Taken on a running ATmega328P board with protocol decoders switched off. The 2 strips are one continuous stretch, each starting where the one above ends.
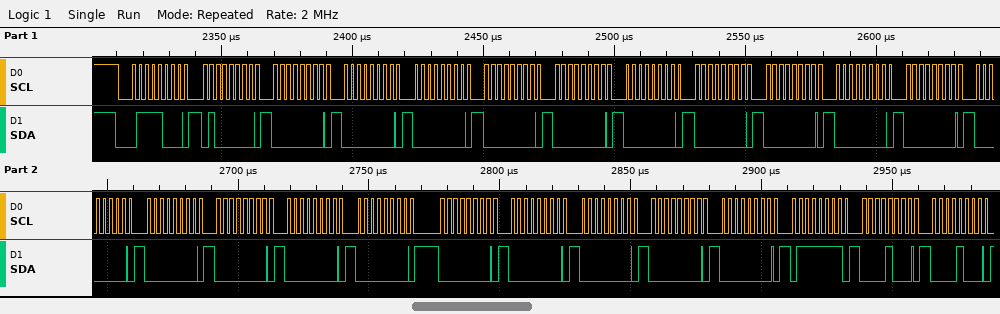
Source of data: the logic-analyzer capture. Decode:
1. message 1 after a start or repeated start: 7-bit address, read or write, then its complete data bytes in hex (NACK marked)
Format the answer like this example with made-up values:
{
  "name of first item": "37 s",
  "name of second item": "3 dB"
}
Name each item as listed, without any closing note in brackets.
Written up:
{
  "message 1 after a start or repeated start: 7-bit address, read or write, then its complete data bytes in hex": "0x3C write: 40 00 00 00 00 00 00 00 00 00 00 00 00 00 00 00 00 00 00 00 00 7F 08 08"
}
